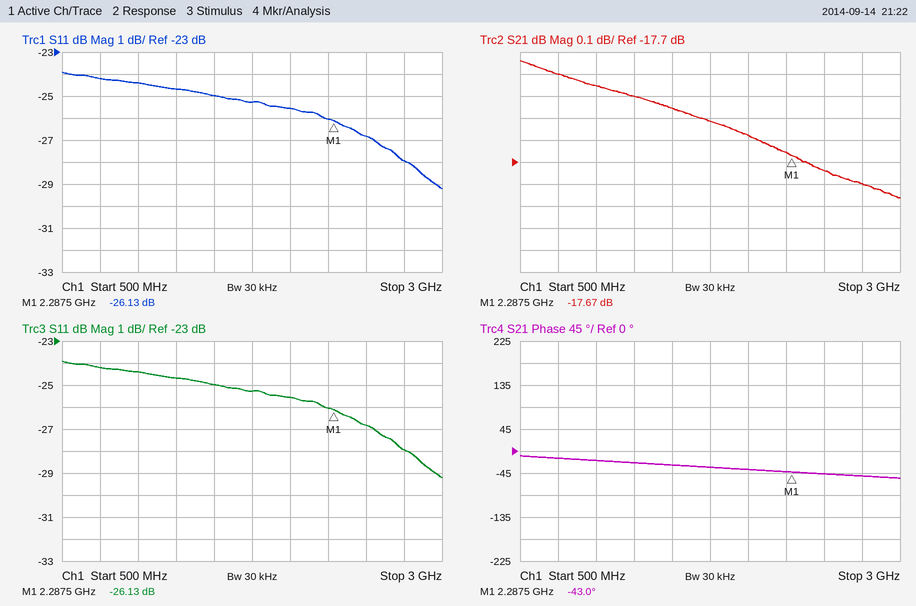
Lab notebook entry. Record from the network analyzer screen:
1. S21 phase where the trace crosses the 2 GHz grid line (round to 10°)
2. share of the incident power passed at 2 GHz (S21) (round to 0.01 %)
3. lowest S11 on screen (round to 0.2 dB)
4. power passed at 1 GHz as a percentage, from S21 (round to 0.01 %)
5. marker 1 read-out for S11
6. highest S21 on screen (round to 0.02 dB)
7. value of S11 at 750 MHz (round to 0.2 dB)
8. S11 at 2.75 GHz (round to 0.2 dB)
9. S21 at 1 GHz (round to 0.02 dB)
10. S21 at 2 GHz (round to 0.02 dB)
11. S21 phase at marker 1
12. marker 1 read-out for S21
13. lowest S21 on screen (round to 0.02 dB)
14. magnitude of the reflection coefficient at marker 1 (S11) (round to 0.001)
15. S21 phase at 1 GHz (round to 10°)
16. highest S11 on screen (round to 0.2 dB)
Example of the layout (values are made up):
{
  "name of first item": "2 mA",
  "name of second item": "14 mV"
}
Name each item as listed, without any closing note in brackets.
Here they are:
{
  "S21 phase where the trace crosses the 2 GHz grid line": "-40°",
  "share of the incident power passed at 2 GHz (S21)": "1.75 %",
  "lowest S11 on screen": "-29.2 dB",
  "power passed at 1 GHz as a percentage, from S21": "1.84 %",
  "marker 1 read-out for S11": "-26.13 dB",
  "highest S21 on screen": "-17.24 dB",
  "value of S11 at 750 MHz": "-24.2 dB",
  "S11 at 2.75 GHz": "-28.0 dB",
  "S21 at 1 GHz": "-17.36 dB",
  "S21 at 2 GHz": "-17.58 dB",
  "S21 phase at marker 1": "-43.0°",
  "marker 1 read-out for S21": "-17.67 dB",
  "lowest S21 on screen": "-17.86 dB",
  "magnitude of the reflection coefficient at marker 1 (S11)": "0.049",
  "S21 phase at 1 GHz": "-20°",
  "highest S11 on screen": "-24.0 dB"
}
